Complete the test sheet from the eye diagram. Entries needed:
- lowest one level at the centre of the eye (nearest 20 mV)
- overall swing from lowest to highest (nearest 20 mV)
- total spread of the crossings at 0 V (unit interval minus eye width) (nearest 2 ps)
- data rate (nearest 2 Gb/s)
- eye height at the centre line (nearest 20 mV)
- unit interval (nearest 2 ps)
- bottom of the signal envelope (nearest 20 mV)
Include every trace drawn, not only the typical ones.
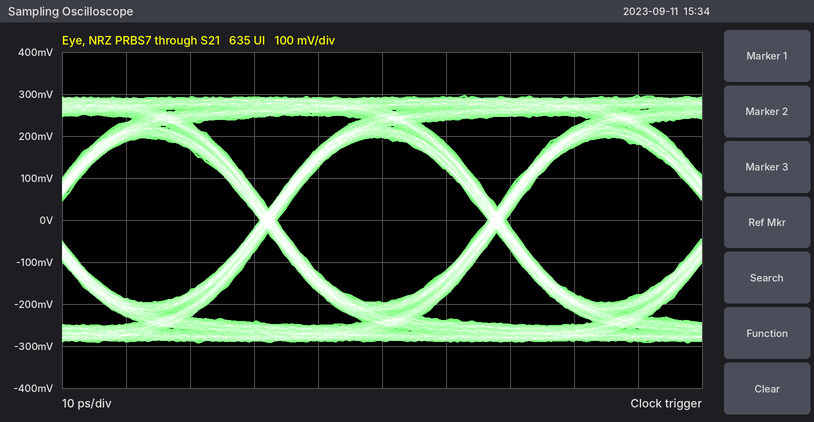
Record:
200 mV
580 mV
2 ps
28 Gb/s
400 mV
36 ps
-300 mV
